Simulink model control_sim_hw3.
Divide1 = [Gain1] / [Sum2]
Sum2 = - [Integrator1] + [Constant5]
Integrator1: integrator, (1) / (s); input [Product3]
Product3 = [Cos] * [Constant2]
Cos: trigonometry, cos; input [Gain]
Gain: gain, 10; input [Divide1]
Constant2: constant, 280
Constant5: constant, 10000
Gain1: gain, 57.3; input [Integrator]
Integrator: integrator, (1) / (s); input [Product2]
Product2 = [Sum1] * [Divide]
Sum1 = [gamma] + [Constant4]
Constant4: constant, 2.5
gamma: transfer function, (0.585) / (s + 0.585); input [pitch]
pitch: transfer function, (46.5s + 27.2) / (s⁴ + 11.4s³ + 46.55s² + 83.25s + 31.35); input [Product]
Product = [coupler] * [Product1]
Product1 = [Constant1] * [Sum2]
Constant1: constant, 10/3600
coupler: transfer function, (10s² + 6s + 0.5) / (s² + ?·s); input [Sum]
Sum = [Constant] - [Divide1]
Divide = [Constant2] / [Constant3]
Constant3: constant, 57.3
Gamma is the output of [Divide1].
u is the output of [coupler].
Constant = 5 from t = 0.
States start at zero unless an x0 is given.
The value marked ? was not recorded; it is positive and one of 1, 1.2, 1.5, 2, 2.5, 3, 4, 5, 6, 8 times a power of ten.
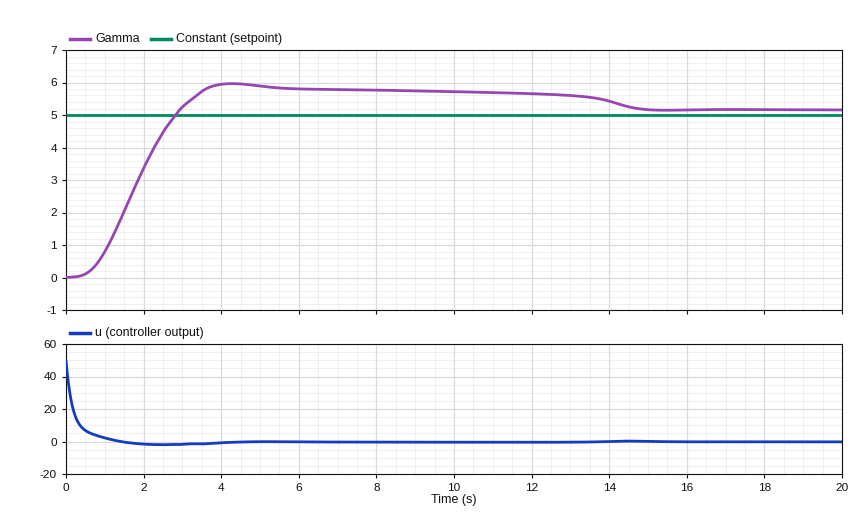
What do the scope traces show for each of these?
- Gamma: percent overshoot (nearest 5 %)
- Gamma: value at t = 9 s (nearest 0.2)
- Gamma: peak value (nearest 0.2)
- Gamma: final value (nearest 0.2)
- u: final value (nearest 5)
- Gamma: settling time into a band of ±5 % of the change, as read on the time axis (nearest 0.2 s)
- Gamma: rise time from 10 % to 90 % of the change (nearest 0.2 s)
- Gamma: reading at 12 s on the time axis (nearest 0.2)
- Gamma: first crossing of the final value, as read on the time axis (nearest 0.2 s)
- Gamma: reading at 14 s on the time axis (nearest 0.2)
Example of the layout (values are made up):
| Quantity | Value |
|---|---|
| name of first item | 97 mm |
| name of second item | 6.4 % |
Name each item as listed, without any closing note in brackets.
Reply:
| Quantity | Value |
|---|---|
| Gamma: percent overshoot | 15 % |
| Gamma: value at t = 9 s | 5.8 |
| Gamma: peak value | 6.0 |
| Gamma: final value | 5.2 |
| u: final value | 0 |
| Gamma: settling time into a band of ±5 % of the change, as read on the time axis | 14.0 s |
| Gamma: rise time from 10 % to 90 % of the change | 1.8 s |
| Gamma: reading at 12 s on the time axis | 5.6 |
| Gamma: first crossing of the final value, as read on the time axis | 3.0 s |
| Gamma: reading at 14 s on the time axis | 5.4 |
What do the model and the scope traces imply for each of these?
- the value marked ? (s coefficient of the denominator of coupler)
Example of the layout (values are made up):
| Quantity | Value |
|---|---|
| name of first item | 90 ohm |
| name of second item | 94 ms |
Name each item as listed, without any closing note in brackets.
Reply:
| Quantity | Value |
|---|---|
| the value marked ? | 6 |
